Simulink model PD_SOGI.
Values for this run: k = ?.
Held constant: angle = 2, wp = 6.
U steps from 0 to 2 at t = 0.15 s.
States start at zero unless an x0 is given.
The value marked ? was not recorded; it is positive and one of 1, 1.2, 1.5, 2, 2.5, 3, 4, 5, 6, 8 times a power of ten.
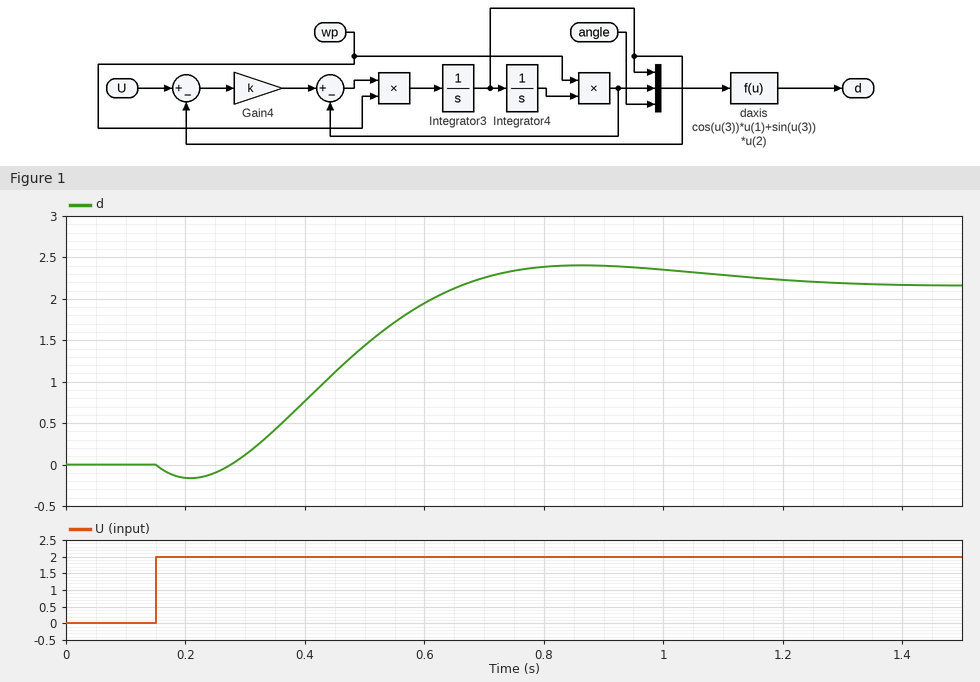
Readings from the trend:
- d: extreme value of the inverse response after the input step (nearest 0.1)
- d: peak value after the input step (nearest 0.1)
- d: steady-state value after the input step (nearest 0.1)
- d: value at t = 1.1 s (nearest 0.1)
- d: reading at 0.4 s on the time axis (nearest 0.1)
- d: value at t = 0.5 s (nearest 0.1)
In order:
-0.2
2.4
2.2
2.3
0.8
1.4
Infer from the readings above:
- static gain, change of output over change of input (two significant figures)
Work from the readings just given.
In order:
1.1
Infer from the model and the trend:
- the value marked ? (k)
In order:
1.2
